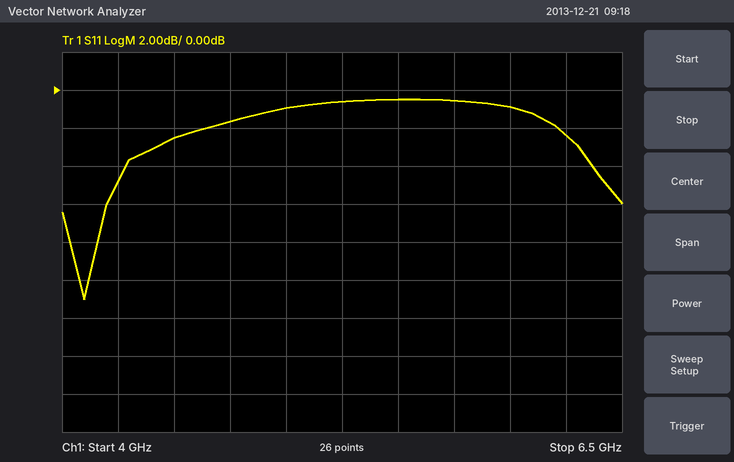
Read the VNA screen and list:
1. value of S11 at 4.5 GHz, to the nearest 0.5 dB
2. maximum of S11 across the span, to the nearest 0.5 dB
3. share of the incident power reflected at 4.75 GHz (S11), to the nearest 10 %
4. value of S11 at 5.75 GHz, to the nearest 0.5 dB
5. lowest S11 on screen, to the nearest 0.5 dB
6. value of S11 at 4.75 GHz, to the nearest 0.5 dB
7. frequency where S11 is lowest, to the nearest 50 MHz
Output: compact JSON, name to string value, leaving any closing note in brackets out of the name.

{"value of S11 at 4.5 GHz, to the nearest 0.5 dB": "-2.5 dB", "maximum of S11 across the span, to the nearest 0.5 dB": "-0.5 dB", "share of the incident power reflected at 4.75 GHz (S11), to the nearest 10 %": "70 %", "value of S11 at 5.75 GHz, to the nearest 0.5 dB": "-0.5 dB", "lowest S11 on screen, to the nearest 0.5 dB": "-11.0 dB", "value of S11 at 4.75 GHz, to the nearest 0.5 dB": "-1.5 dB", "frequency where S11 is lowest, to the nearest 50 MHz": "4.10 GHz"}
